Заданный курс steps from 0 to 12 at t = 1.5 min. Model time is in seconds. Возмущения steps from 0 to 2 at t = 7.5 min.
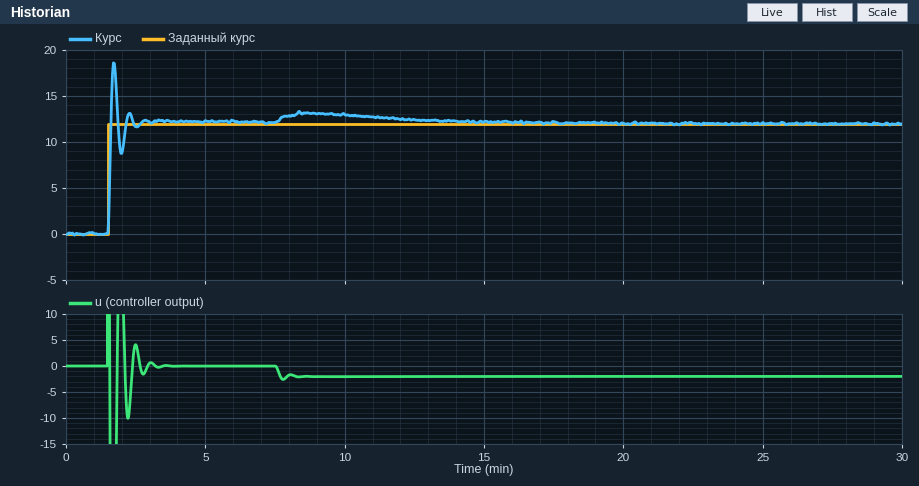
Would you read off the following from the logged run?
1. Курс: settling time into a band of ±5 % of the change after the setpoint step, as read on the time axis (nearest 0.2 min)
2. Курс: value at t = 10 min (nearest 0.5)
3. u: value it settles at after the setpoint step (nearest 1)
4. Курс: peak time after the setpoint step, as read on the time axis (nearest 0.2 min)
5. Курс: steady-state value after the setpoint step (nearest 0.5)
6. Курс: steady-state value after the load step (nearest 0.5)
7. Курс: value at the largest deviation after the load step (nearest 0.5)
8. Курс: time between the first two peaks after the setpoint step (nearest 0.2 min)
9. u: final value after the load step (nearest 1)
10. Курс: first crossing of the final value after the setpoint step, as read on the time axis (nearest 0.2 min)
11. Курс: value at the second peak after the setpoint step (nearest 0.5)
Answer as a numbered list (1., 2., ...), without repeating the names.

1. 2.4 min
2. 13.0
3. 0
4. 1.8 min
5. 12.0
6. 12.0
7. 13.0
8. 0.6 min
9. -2
10. 1.6 min
11. 13.0
